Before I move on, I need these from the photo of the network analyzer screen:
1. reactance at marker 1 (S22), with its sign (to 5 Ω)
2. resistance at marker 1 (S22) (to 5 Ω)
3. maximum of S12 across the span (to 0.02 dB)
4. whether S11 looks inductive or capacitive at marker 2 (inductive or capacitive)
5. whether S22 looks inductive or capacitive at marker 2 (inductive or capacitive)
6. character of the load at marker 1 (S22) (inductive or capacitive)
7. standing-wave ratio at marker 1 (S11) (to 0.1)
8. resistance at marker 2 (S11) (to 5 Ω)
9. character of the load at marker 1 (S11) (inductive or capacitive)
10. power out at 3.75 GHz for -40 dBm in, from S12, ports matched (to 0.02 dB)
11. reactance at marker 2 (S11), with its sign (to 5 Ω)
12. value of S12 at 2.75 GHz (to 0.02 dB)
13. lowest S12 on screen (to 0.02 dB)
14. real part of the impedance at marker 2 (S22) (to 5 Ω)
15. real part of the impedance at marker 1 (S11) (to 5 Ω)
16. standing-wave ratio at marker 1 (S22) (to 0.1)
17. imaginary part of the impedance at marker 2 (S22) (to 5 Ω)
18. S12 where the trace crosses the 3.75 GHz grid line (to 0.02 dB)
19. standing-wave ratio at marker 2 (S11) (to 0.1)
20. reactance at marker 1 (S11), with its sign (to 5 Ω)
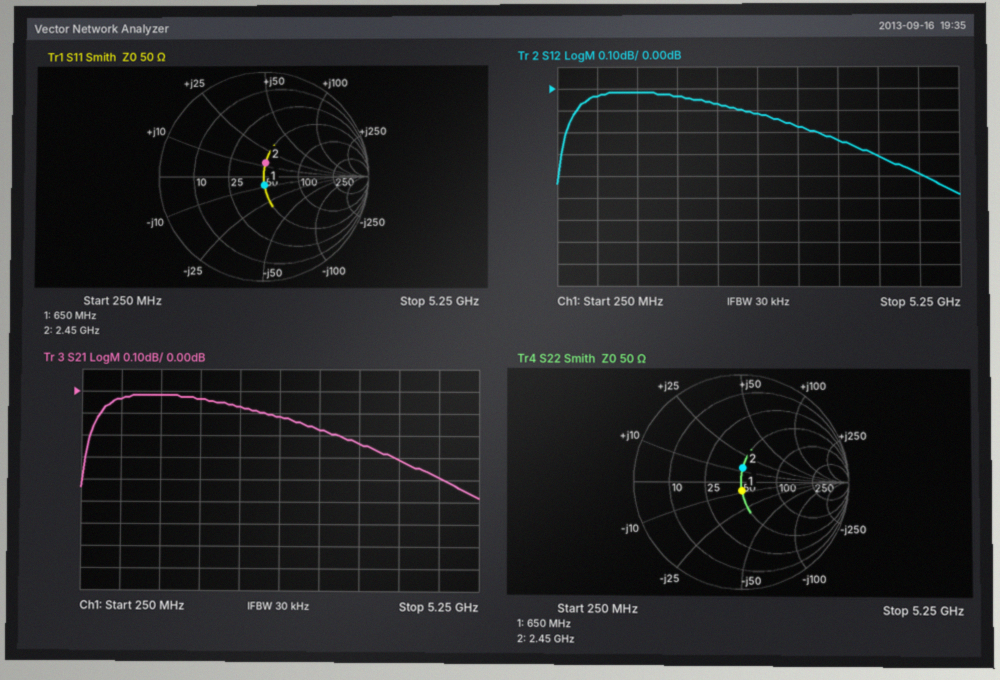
-10 Ω
50 Ω
-0.02 dB
inductive
inductive
capacitive
1.2
50 Ω
capacitive
-40.24 dBm
+15 Ω
-0.12 dB
-0.48 dB
50 Ω
50 Ω
1.2
+15 Ω
-0.24 dB
1.3
-10 Ω
